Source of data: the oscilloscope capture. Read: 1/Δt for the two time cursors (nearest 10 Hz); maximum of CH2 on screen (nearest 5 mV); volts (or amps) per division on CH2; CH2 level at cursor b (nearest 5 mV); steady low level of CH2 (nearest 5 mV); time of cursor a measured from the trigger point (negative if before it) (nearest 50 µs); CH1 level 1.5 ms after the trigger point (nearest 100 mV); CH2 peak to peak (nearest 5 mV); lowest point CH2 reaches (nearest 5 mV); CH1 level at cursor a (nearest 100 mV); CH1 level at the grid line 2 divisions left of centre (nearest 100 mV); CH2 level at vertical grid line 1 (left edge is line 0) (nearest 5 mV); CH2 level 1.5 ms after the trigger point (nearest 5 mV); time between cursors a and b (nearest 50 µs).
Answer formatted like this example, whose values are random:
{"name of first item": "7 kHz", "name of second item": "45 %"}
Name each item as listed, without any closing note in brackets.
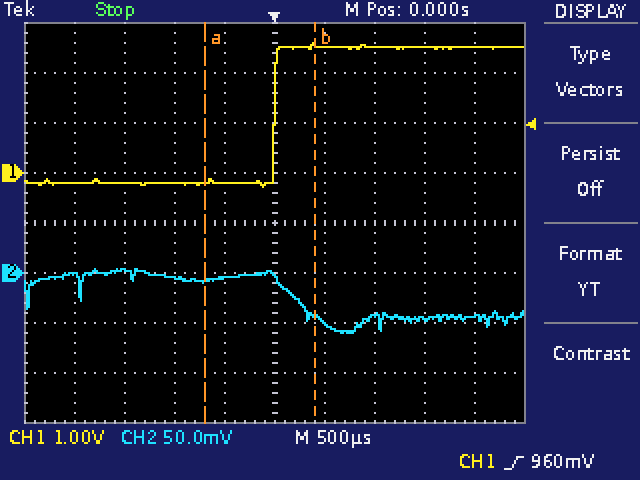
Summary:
{"1/Δt for the two time cursors": "910 Hz", "maximum of CH2 on screen": "5 mV", "volts (or amps) per division on CH2": "50 mV", "CH2 level at cursor b": "-45 mV", "steady low level of CH2": "-45 mV", "time of cursor a measured from the trigger point (negative if before it)": "-700 µs", "CH1 level 1.5 ms after the trigger point": "2.5 V", "CH2 peak to peak": "65 mV", "lowest point CH2 reaches": "-60 mV", "CH1 level at cursor a": "-200 mV", "CH1 level at the grid line 2 divisions left of centre": "-200 mV", "CH2 level at vertical grid line 1 (left edge is line 0)": "0 mV", "CH2 level 1.5 ms after the trigger point": "-45 mV", "time between cursors a and b": "1.10 ms"}
